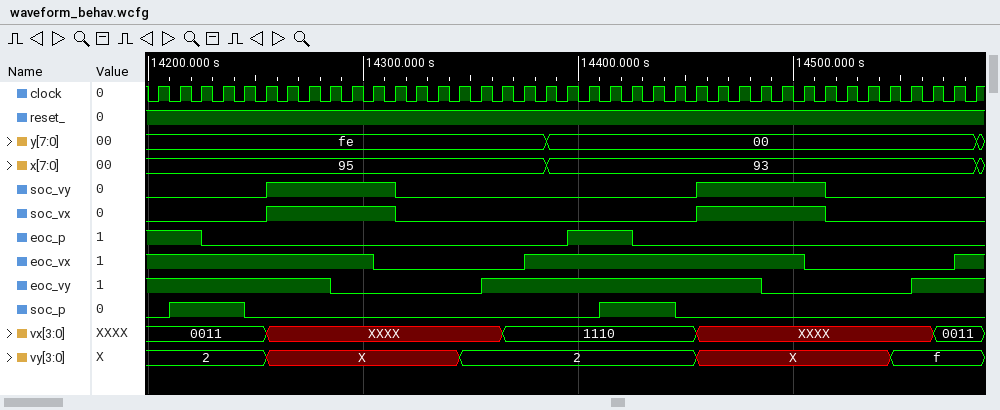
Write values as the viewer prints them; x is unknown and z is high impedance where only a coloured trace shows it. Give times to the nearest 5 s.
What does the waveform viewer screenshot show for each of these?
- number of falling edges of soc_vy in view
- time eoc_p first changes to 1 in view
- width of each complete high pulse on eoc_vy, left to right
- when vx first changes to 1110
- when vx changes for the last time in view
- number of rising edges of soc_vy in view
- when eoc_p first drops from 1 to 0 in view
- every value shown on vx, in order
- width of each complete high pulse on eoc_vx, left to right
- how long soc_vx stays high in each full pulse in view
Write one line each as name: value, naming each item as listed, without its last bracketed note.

number of falling edges of soc_vy in view: 2
time eoc_p first changes to 1 in view: 14395 s
width of each complete high pulse on eoc_vy, left to right: 130 s
when vx first changes to 1110: 14365 s
when vx changes for the last time in view: 14565 s
number of rising edges of soc_vy in view: 2
when eoc_p first drops from 1 to 0 in view: 14225 s
every value shown on vx, in order: 0011, XXXX, 1110, XXXX, 0011
width of each complete high pulse on eoc_vx, left to right: 130 s
how long soc_vx stays high in each full pulse in view: 60 s, 60 s
